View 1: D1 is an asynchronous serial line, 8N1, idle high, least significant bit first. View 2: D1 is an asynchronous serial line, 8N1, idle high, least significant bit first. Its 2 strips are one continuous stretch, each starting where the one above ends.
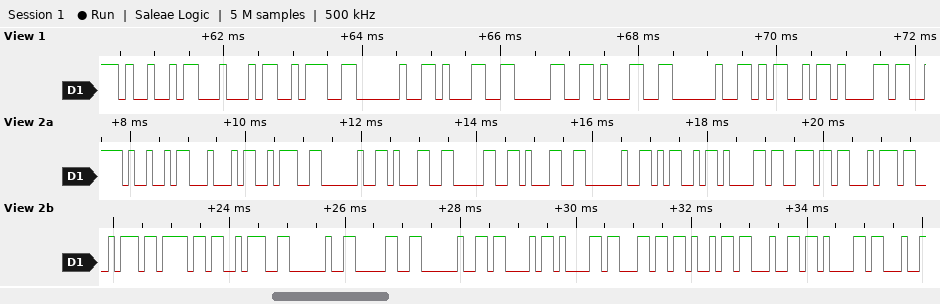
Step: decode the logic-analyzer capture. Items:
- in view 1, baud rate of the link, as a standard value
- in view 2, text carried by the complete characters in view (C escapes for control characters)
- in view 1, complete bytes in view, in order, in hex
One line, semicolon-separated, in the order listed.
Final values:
9600 baud; "ID: 101 Mantto: 0 Calida"; 0x49 0x44 0x3A 0x20 0x31 0x30 0x31 0x20 0x4D 0x61
